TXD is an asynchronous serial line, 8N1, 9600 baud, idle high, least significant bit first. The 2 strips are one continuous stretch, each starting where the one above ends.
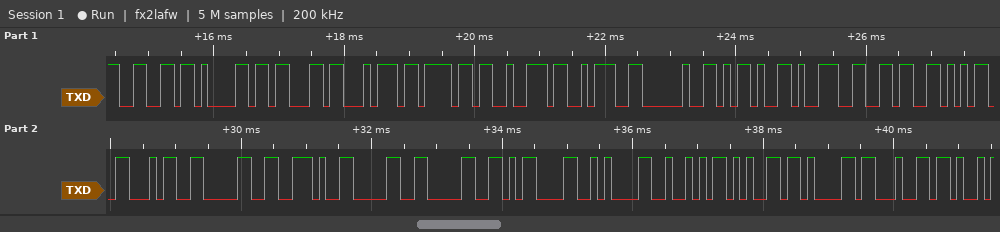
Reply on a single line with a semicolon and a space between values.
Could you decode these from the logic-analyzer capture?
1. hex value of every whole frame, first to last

66 61 63 74 6F 72 3A 20 2D 39 36 35 34 30 2E 30 30 0D 0A 52 65 61 64
